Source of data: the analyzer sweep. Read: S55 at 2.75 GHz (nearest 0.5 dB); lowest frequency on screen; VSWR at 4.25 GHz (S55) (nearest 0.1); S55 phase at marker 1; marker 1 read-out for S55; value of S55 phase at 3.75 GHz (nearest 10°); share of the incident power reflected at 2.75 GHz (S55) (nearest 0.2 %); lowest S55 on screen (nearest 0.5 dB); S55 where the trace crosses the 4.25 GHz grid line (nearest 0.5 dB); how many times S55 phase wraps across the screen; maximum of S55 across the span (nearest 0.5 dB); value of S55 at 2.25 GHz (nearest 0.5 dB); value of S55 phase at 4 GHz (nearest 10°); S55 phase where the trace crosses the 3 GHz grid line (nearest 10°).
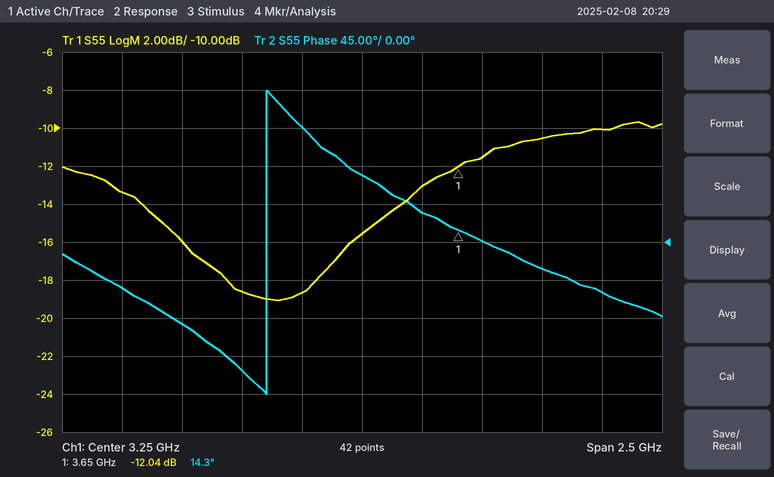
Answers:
-18.5 dB
2 GHz
1.9
14.3°
-12.04 dB
0°
1.4 %
-19.0 dB
-10.0 dB
1
-9.5 dB
-13.5 dB
-30°
140°
